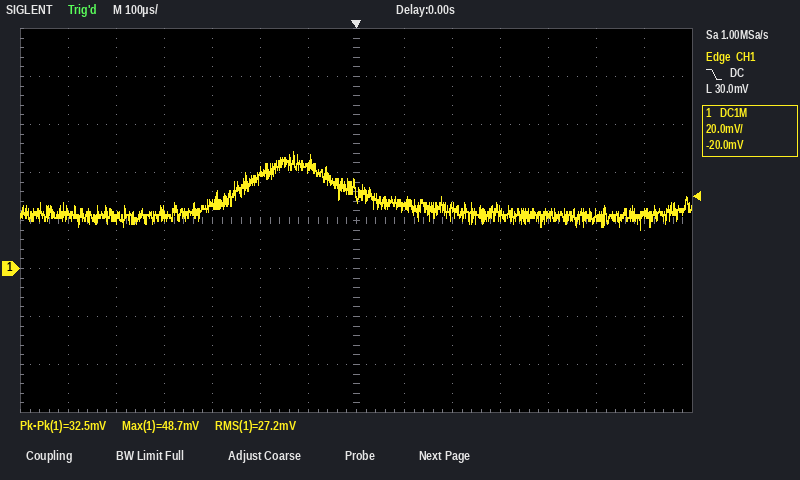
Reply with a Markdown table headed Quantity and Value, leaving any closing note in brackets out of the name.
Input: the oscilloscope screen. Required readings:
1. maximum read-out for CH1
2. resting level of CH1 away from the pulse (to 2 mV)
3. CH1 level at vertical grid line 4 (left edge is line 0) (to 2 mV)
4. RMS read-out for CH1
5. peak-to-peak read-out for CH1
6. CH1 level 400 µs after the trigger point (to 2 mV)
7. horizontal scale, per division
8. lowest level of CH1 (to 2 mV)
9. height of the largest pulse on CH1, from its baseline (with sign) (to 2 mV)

| Quantity | Value |
|---|---|
| maximum read-out for CH1 | 48.7 mV |
| resting level of CH1 away from the pulse | 22 mV |
| CH1 level at vertical grid line 4 (left edge is line 0) | 26 mV |
| RMS read-out for CH1 | 27.2 mV |
| peak-to-peak read-out for CH1 | 32.5 mV |
| CH1 level 400 µs after the trigger point | 22 mV |
| horizontal scale, per division | 100 µs |
| lowest level of CH1 | 16 mV |
| height of the largest pulse on CH1, from its baseline (with sign) | +26 mV |
